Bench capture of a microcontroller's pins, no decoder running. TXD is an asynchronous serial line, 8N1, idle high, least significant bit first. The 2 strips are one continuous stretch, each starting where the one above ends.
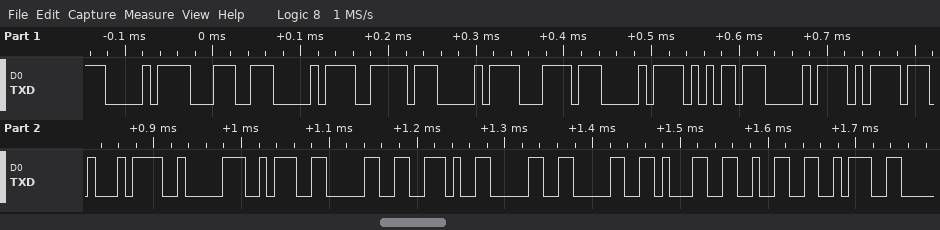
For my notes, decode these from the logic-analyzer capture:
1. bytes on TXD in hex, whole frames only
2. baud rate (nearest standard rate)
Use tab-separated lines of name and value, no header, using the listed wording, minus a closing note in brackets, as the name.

bytes on TXD in hex, whole frames only	D0 9C D0 BE D0 BC D0 B5 D0 BD D1 82 3A 30 2E 30 30 31 32 3A
baud rate	115200 baud
